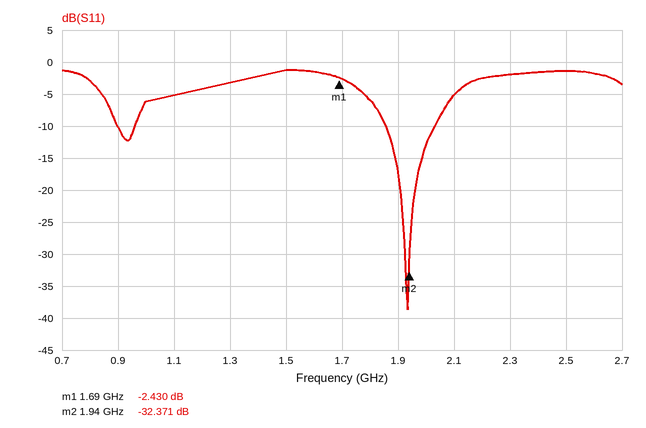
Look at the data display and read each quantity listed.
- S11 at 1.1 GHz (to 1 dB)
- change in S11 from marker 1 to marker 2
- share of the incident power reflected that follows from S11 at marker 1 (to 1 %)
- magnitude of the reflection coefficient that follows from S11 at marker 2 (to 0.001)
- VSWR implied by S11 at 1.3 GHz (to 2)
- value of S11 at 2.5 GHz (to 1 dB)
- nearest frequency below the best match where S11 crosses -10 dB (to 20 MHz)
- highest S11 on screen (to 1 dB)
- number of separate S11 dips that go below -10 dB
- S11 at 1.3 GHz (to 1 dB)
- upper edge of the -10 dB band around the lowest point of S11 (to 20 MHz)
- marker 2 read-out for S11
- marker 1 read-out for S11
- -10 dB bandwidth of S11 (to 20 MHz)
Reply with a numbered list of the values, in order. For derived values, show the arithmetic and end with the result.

1. -5 dB
2. -32.371 − (-2.43) = -29.941 dB
3. 10^(-2.43/10) ≈ 57 %
4. 10^(-32.371/20) ≈ 0.024
5. |Γ| = 10^(-3/20) = 0.7079; VSWR = (1 + 0.7079)/(1 − 0.7079) ≈ 6
6. -1 dB
7. 1.86 GHz
8. -1 dB
9. 2
10. -3 dB
11. 2.04 GHz
12. -32.371 dB
13. -2.430 dB
14. 2.04 GHz − 1.86 GHz = 180 MHz
